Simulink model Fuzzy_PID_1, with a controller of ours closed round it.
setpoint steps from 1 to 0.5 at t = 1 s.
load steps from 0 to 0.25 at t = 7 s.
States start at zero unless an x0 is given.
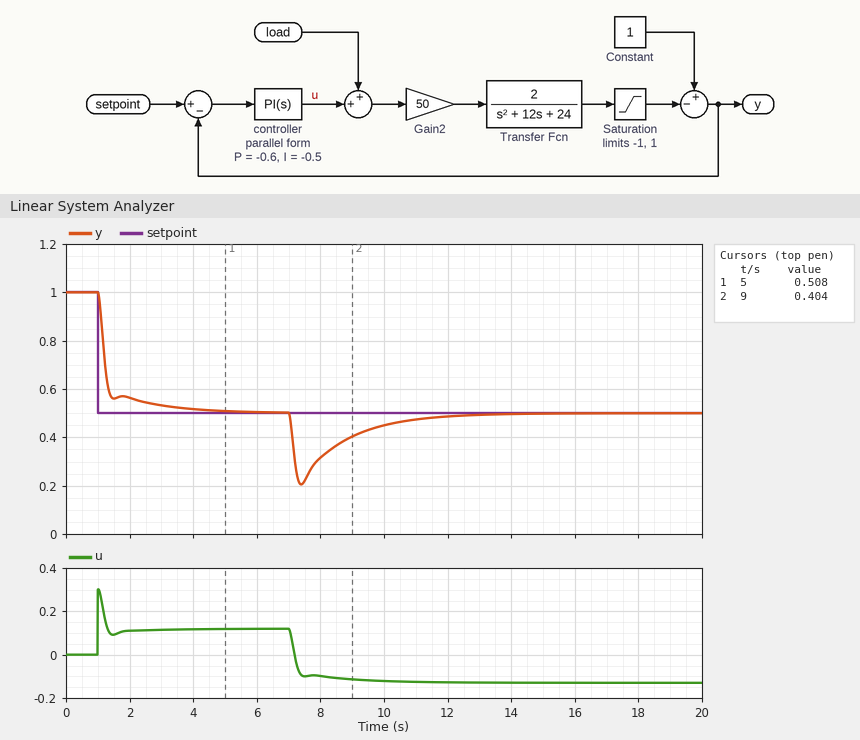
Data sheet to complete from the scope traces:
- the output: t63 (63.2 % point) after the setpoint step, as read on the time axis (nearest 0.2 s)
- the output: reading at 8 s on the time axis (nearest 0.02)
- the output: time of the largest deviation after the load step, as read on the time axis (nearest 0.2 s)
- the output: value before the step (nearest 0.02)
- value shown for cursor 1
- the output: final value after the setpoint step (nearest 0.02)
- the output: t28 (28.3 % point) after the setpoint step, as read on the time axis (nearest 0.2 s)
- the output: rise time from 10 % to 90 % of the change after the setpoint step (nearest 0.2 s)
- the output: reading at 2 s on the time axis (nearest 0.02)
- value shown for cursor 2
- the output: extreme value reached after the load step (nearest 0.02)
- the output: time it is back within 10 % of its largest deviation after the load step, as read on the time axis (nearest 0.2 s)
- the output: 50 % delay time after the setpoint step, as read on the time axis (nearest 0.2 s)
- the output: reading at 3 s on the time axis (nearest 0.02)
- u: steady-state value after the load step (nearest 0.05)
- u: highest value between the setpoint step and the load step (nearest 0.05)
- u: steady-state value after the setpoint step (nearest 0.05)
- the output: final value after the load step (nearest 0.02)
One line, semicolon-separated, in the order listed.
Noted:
1.2 s; 0.32; 7.4 s; 1.00; 0.508; 0.50; 1.2 s; 1.2 s; 0.56; 0.404; 0.20; 10.8 s; 1.2 s; 0.54; -0.15; 0.30; 0.10; 0.50
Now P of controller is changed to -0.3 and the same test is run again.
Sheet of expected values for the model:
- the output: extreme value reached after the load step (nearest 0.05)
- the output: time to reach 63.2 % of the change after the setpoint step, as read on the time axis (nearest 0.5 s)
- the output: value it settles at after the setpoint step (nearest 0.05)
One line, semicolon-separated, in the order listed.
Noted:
0.10; 1.5 s; 0.50
